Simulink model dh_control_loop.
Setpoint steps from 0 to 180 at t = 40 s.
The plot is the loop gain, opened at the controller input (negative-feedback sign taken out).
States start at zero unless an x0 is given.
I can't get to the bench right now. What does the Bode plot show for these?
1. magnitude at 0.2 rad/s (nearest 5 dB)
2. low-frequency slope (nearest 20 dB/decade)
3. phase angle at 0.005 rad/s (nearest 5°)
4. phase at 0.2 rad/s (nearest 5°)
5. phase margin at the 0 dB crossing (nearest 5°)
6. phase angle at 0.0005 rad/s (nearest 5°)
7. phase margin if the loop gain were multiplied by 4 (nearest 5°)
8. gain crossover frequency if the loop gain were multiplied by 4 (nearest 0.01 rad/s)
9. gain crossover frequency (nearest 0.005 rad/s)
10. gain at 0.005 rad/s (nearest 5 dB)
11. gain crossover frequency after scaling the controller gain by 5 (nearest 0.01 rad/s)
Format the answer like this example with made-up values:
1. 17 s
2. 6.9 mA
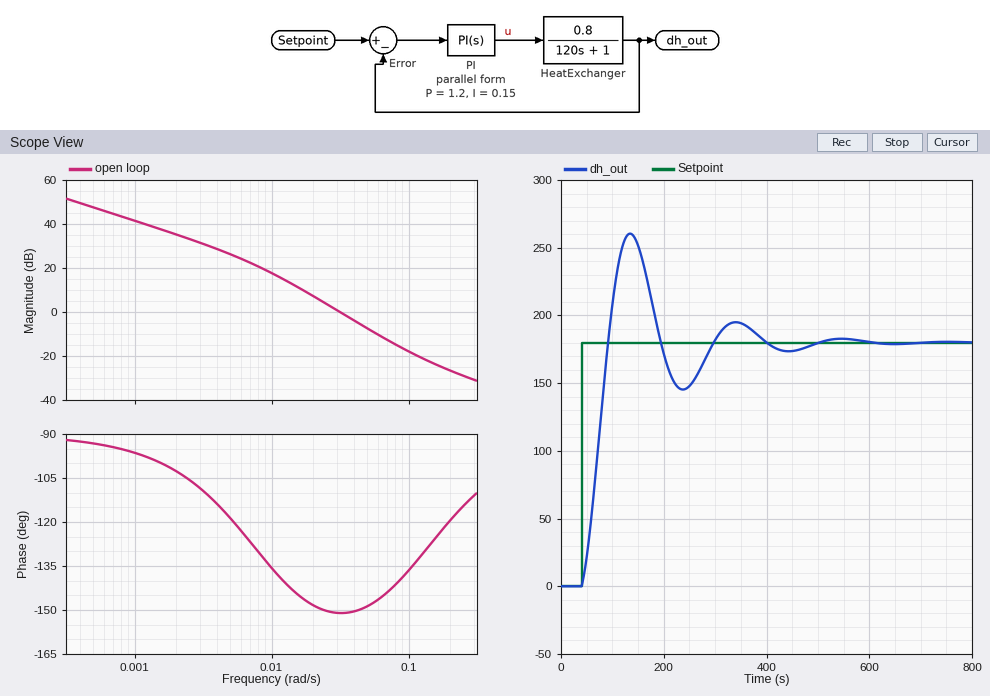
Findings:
1. -25 dB
2. -20 dB/decade
3. -120°
4. -120°
5. 30°
6. -95°
7. 35°
8. 0.07 rad/s
9. 0.030 rad/s
10. 25 dB
11. 0.08 rad/s
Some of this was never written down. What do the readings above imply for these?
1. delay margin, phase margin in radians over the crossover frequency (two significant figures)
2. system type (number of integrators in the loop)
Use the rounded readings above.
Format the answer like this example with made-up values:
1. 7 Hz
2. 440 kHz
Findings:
1. 17 s
2. 1
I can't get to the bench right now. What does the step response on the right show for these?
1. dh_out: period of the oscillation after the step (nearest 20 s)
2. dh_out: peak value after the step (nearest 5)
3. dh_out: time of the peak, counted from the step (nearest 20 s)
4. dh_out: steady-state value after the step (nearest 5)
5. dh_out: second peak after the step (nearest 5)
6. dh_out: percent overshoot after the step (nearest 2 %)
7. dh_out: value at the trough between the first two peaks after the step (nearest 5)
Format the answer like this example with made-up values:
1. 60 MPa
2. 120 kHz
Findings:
1. 200 s
2. 260
3. 100 s
4. 180
5. 195
6. 44 %
7. 145
